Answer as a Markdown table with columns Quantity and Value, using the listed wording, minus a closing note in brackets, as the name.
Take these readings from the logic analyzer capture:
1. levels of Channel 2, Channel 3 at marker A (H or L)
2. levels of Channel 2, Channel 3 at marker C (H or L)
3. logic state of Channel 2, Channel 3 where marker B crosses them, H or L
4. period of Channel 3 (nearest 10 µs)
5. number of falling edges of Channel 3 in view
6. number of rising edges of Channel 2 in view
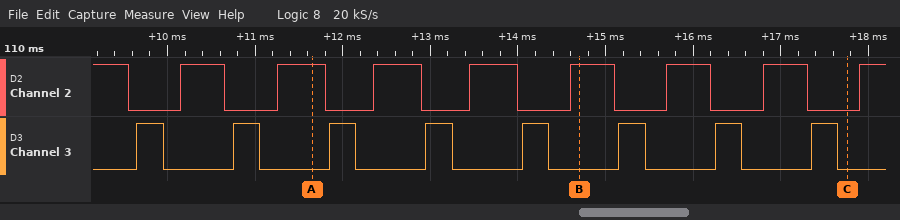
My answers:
| Quantity | Value |
|---|---|
| levels of Channel 2, Channel 3 at marker A | Channel 2=H, Channel 3=L |
| levels of Channel 2, Channel 3 at marker C | Channel 2=L, Channel 3=L |
| logic state of Channel 2, Channel 3 where marker B crosses them, H or L | Channel 2=H, Channel 3=L |
| period of Channel 3 | 1100 µs |
| number of falling edges of Channel 3 in view | 8 |
| number of rising edges of Channel 2 in view | 8 |
